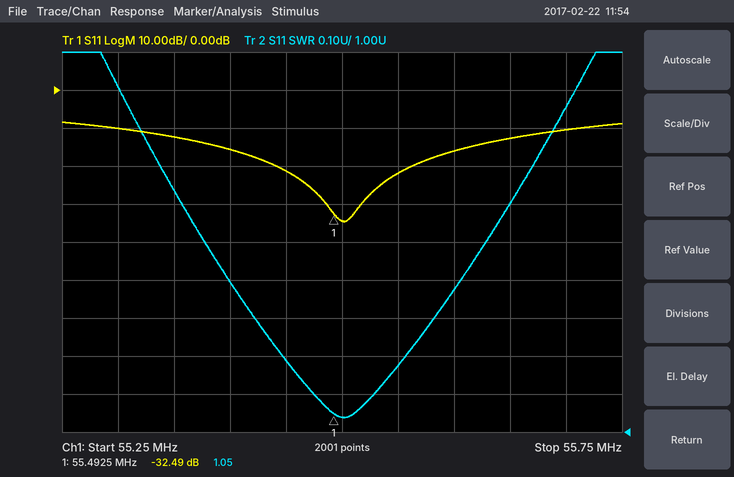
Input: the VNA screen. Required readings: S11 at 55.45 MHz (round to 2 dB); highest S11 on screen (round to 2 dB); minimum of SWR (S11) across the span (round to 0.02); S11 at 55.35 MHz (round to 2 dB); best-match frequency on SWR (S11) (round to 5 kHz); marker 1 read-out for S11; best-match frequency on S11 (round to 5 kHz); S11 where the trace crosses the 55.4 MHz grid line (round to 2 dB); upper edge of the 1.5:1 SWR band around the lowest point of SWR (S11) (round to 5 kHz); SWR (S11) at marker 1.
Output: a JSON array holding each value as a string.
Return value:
["-22 dB", "-8 dB", "1.04", "-12 dB", "55.500 MHz", "-32.49 dB", "55.500 MHz", "-16 dB", "55.630 MHz", "1.05"]
